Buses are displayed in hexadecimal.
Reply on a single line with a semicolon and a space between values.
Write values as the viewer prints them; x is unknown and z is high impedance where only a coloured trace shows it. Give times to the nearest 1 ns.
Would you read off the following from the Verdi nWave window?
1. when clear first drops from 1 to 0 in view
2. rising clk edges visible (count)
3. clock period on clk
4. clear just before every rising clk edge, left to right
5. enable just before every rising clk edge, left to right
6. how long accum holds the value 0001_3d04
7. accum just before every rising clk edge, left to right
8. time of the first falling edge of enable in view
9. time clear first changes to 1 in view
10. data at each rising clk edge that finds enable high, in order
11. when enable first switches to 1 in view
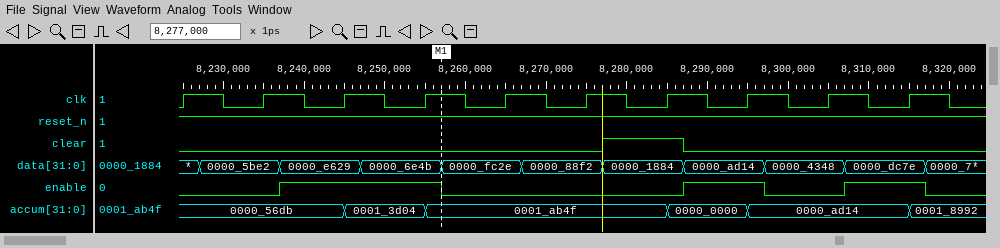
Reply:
8287 ns; 10; 10 ns; 0 0 0 0 0 0 1 0 0 0; 0 0 1 1 0 0 0 1 0 1; 10 ns; 0000_56db, 0000_56db, 0000_56db, 0001_3d04, 0001_ab4f, 0001_ab4f, 0001_ab4f, 0000_0000, 0000_ad14, 0000_ad14; 8257 ns; 8277 ns; 0000_e629, 0000_6e4b, 0000_ad14, 0000_dc7e; 8237 ns
